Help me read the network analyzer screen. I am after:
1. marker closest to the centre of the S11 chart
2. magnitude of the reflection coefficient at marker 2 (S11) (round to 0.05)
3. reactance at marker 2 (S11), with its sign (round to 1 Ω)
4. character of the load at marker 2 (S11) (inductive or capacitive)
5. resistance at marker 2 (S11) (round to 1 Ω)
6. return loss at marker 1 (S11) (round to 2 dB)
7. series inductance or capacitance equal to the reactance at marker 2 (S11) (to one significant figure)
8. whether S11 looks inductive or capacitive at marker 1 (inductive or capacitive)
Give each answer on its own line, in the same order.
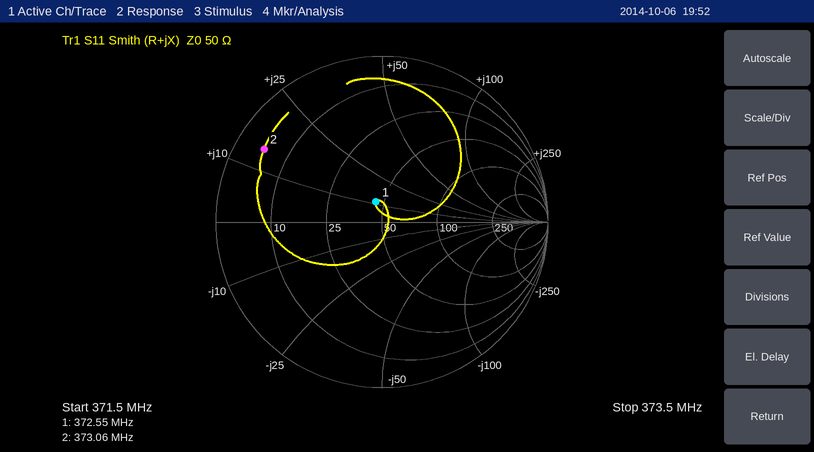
marker 1
0.85
+14 Ω
inductive
5 Ω
18 dB
6 nH
inductive
